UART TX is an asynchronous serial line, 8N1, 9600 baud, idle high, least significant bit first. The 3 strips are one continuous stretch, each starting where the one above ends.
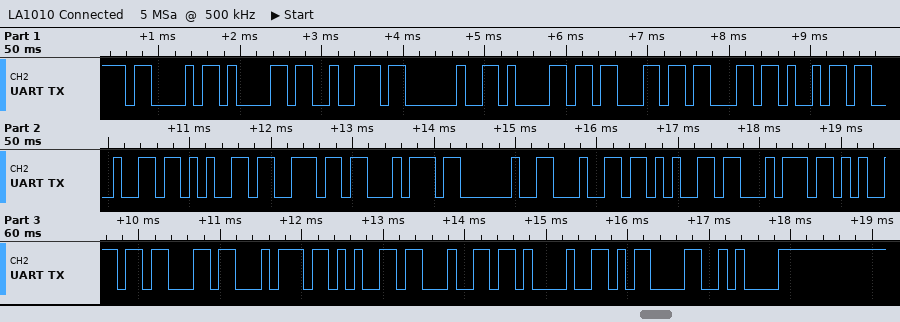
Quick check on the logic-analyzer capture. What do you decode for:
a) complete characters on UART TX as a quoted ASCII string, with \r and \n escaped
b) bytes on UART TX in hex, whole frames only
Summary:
"Car accident detected!\r\n"
0x43 0x61 0x72 0x20 0x61 0x63 0x63 0x69 0x64 0x65 0x6E 0x74 0x20 0x64 0x65 0x74 0x65 0x63 0x74 0x65 0x64 0x21 0x0D 0x0A
